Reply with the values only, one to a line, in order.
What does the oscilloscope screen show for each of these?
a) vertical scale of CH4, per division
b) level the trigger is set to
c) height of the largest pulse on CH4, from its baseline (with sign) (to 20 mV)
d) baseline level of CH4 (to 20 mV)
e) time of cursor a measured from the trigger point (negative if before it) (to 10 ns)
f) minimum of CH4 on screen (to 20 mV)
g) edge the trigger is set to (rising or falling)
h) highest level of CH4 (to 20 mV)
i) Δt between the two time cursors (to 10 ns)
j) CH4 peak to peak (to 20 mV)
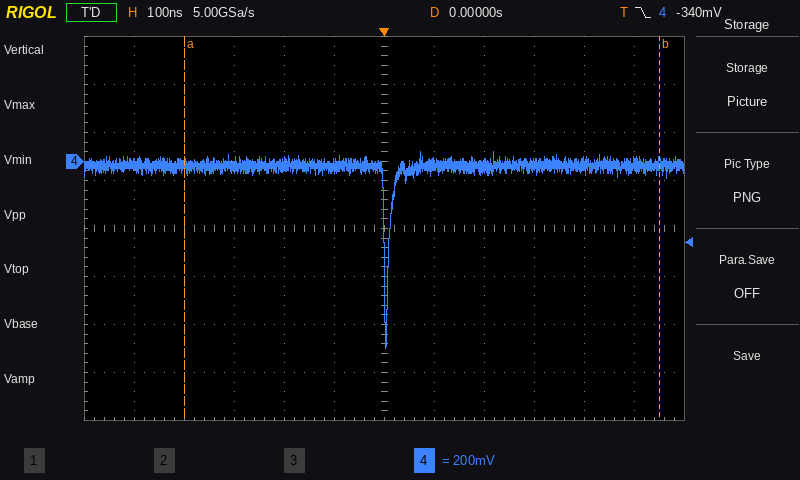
200 mV
-340 mV
-760 mV
-20 mV
-400 ns
-780 mV
falling
40 mV
950 ns
820 mV
